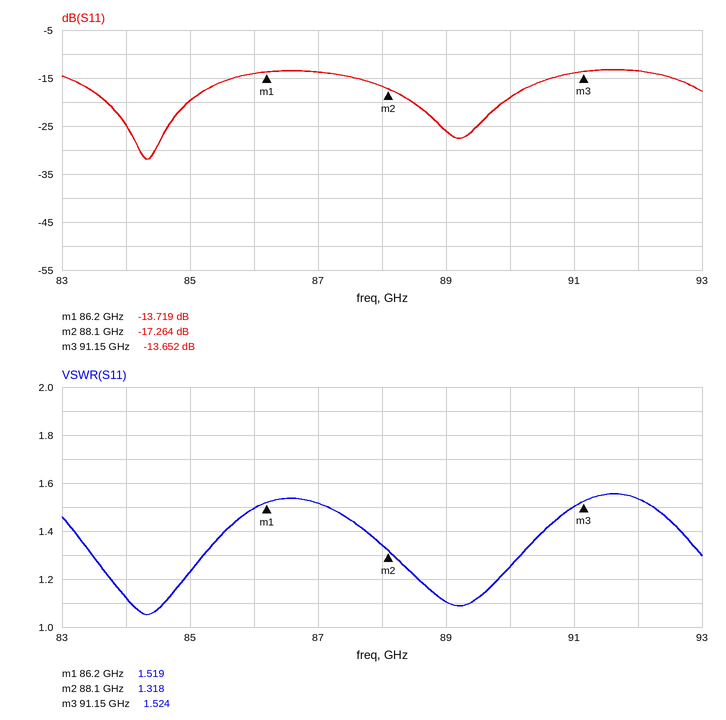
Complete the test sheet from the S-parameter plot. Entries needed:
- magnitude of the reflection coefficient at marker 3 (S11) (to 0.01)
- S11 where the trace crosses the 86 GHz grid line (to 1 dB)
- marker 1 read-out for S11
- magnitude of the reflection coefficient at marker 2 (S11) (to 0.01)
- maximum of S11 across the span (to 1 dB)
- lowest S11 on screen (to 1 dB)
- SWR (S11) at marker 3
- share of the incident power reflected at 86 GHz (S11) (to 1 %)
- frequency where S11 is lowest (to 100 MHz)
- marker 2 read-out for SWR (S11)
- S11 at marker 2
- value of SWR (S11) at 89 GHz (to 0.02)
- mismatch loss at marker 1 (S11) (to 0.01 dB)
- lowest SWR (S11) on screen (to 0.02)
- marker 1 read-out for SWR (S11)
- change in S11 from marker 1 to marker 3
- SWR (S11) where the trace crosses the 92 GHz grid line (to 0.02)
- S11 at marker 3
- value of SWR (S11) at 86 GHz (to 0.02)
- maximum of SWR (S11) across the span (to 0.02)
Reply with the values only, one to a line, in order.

0.21
-14 dB
-13.719 dB
0.14
-13 dB
-32 dB
1.524
4 %
84.3 GHz
1.318
-17.264 dB
1.10
0.19 dB
1.06
1.519
0.067 dB
1.54
-13.652 dB
1.50
1.56
